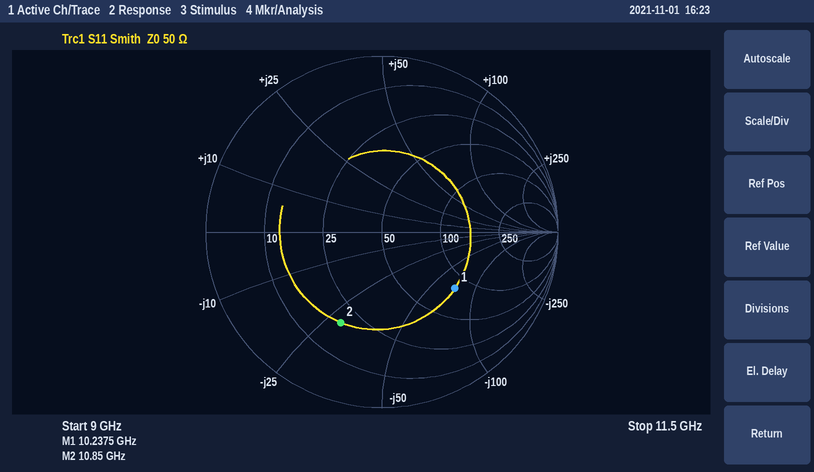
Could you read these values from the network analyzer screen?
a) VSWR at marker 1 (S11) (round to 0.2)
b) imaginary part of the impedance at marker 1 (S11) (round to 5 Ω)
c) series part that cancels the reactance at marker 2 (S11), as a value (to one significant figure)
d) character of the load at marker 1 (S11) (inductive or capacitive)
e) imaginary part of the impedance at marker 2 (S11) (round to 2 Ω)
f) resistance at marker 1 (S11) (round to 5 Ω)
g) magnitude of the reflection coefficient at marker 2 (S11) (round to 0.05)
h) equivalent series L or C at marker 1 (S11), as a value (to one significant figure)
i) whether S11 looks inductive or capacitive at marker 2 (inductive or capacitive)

3.2
-70 Ω
400 pH
capacitive
-28 Ω
80 Ω
0.55
200 fF
capacitive
